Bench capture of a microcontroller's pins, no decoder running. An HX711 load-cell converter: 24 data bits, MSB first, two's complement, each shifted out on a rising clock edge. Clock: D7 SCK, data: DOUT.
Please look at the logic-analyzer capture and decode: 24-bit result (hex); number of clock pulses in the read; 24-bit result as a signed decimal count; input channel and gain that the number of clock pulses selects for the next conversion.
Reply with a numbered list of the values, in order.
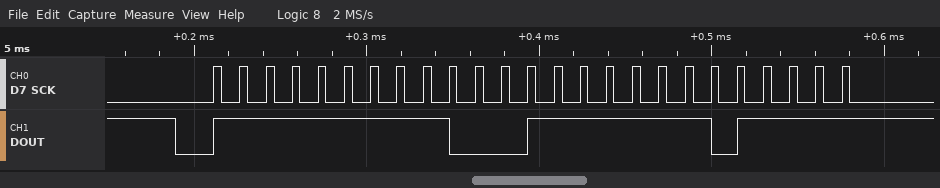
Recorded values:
1. 0xFF8FEF
2. 25
3. -28689
4. channel A, gain 128
